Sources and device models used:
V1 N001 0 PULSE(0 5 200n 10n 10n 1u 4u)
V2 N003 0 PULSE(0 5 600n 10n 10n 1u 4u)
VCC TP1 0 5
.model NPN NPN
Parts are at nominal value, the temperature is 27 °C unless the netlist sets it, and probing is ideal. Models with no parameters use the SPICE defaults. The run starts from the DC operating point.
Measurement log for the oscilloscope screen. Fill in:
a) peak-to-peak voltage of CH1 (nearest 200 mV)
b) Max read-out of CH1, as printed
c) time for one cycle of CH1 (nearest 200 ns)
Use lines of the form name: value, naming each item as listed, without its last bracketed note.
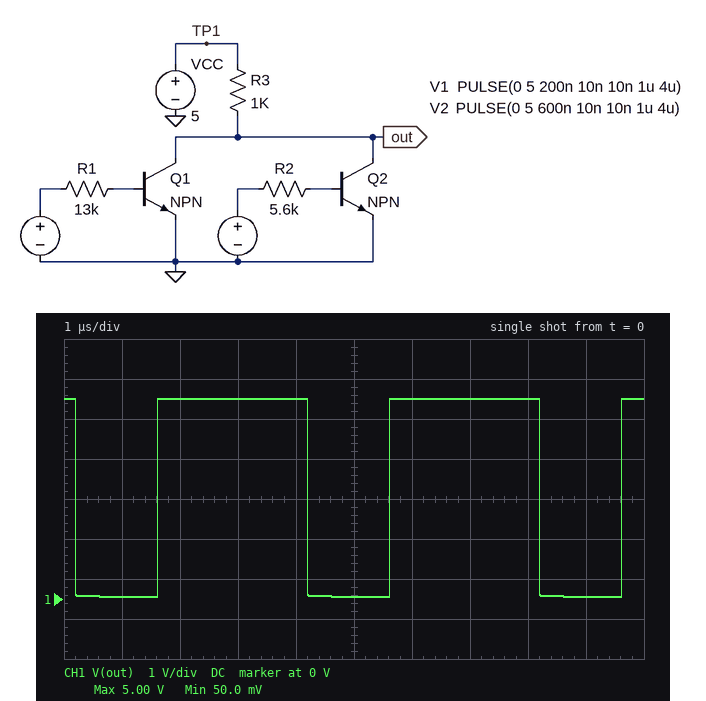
peak-to-peak voltage of CH1: 5.0 V
Max read-out of CH1, as printed: 5.00 V
time for one cycle of CH1: 4.0 µs
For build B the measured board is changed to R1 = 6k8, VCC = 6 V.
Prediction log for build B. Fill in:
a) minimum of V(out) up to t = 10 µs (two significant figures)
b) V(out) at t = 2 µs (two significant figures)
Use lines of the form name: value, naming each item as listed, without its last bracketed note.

minimum of V(out) up to t = 10 µs: 49 mV
V(out) at t = 2 µs: 6.0 V
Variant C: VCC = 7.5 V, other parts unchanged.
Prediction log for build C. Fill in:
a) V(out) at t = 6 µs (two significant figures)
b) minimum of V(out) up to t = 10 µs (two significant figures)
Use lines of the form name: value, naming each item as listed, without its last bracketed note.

V(out) at t = 6 µs: 7.5 V
minimum of V(out) up to t = 10 µs: 59 mV
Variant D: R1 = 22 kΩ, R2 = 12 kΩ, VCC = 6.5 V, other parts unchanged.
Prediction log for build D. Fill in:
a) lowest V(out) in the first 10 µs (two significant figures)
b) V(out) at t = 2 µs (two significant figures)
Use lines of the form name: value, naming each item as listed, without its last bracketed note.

lowest V(out) in the first 10 µs: 71 mV
V(out) at t = 2 µs: 6.5 V
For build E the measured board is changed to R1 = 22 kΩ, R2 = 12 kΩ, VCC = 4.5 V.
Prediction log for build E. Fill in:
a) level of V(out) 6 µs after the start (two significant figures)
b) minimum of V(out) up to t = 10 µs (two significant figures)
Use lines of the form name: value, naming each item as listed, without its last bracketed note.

level of V(out) 6 µs after the start: 4.5 V
minimum of V(out) up to t = 10 µs: 62 mV
